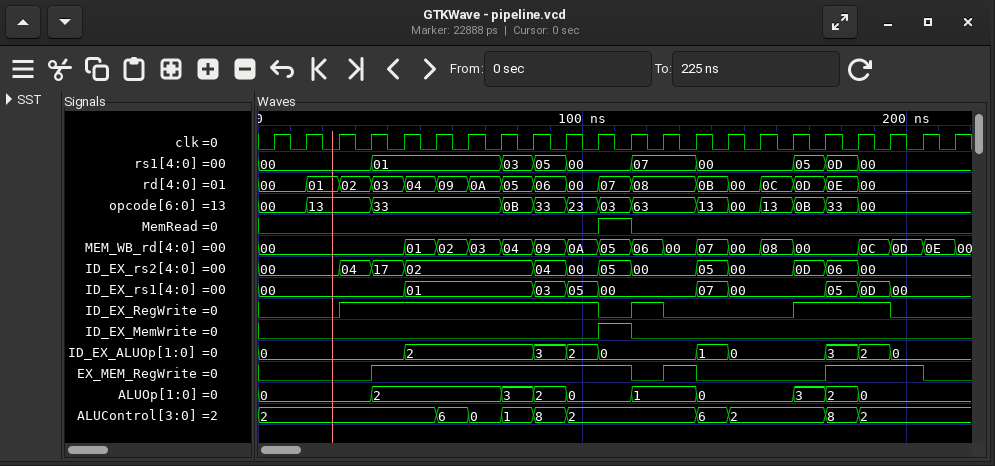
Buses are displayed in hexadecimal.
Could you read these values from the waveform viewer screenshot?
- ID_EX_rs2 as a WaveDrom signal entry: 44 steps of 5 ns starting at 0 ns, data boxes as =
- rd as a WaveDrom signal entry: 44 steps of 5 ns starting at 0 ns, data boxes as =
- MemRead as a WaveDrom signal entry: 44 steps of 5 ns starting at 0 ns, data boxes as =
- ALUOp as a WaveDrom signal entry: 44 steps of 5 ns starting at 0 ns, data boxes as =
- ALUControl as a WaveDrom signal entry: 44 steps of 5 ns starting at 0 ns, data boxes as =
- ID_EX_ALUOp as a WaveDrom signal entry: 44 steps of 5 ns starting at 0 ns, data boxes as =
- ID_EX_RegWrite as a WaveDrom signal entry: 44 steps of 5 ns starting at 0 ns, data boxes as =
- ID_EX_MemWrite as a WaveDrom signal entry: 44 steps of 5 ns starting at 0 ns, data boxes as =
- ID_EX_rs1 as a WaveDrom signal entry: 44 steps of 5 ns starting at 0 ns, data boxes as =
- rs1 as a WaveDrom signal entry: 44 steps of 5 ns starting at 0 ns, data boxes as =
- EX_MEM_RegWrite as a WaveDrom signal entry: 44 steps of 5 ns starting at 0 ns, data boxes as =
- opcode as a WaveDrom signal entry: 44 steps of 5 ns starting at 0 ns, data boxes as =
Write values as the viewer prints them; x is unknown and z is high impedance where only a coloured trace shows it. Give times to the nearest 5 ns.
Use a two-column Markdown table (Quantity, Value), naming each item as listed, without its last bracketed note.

| Quantity | Value |
|---|---|
| ID_EX_rs2 as a WaveDrom signal entry: 44 steps of 5 ns starting at 0 ns, data boxes as = | {name: 'ID_EX_rs2', wave: '=....=.=.=.......=.=.=.=...=.=...=.=.=......', data: '00 04 17 02 04 00 05 00 05 00 0D 06 00'} |
| rd as a WaveDrom signal entry: 44 steps of 5 ns starting at 0 ns, data boxes as = | {name: 'rd', wave: '=..=.=.=.=.=.=.=.=.=.=.=...=.=.=.=.=.=......', data: '00 01 02 03 04 09 0A 05 06 00 07 08 0B 00 0C 0D 0E 00'} |
| MemRead as a WaveDrom signal entry: 44 steps of 5 ns starting at 0 ns, data boxes as = | {name: 'MemRead', wave: '0....................1.0....................'} |
| ALUOp as a WaveDrom signal entry: 44 steps of 5 ns starting at 0 ns, data boxes as = | {name: 'ALUOp', wave: '=......=.......=.=.=...=...=.....=.=.=......', data: '0 2 3 2 0 1 0 3 2 0'} |
| ALUControl as a WaveDrom signal entry: 44 steps of 5 ns starting at 0 ns, data boxes as = | {name: 'ALUControl', wave: '=..........=.=.=.=.=.......=.=.....=.=......', data: '2 6 0 1 8 2 6 2 8 2'} |
| ID_EX_ALUOp as a WaveDrom signal entry: 44 steps of 5 ns starting at 0 ns, data boxes as = | {name: 'ID_EX_ALUOp', wave: '=........=.......=.=.=.....=.=.....=.=.=....', data: '0 2 3 2 0 1 0 3 2 0'} |
| ID_EX_RegWrite as a WaveDrom signal entry: 44 steps of 5 ns starting at 0 ns, data boxes as = | {name: 'ID_EX_RegWrite', wave: '0....1...............0.1.0.......1.....0....'} |
| ID_EX_MemWrite as a WaveDrom signal entry: 44 steps of 5 ns starting at 0 ns, data boxes as = | {name: 'ID_EX_MemWrite', wave: '0....................1.0....................'} |
| ID_EX_rs1 as a WaveDrom signal entry: 44 steps of 5 ns starting at 0 ns, data boxes as = | {name: 'ID_EX_rs1', wave: '=........=.......=.=.=.....=.=.....=.=.=....', data: '00 01 03 05 00 07 00 05 0D 00'} |
| rs1 as a WaveDrom signal entry: 44 steps of 5 ns starting at 0 ns, data boxes as = | {name: 'rs1', wave: '=......=.......=.=.=...=...=.....=.=.=......', data: '00 01 03 05 00 07 00 05 0D 00'} |
| EX_MEM_RegWrite as a WaveDrom signal entry: 44 steps of 5 ns starting at 0 ns, data boxes as = | {name: 'EX_MEM_RegWrite', wave: '0......1...............0.1.0.......1.....0..'} |
| opcode as a WaveDrom signal entry: 44 steps of 5 ns starting at 0 ns, data boxes as = | {name: 'opcode', wave: '=..=...=.......=.=.=.=.=...=.=.=.=.=.=......', data: '00 13 33 0B 33 23 03 63 13 00 13 0B 33 00'} |
